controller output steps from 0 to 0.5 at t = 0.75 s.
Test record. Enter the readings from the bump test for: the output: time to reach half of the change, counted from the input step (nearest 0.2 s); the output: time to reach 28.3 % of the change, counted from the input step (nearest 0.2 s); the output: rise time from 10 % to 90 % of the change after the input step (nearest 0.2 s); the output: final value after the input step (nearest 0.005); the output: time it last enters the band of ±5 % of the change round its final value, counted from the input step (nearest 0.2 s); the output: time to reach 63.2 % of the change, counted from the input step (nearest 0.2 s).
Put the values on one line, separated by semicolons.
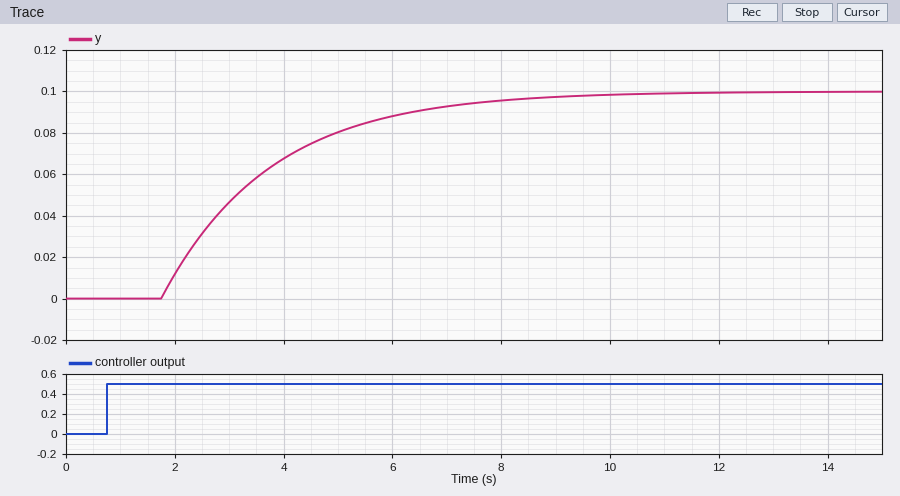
2.4 s; 1.6 s; 4.4 s; 0.100; 7.0 s; 3.0 s
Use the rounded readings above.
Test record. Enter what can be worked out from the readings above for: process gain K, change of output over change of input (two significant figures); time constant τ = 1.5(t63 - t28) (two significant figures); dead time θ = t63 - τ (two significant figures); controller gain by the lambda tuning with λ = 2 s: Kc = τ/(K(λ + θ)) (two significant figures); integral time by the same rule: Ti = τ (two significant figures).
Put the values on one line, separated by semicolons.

0.20; 2.1 s; 0.90 s; 3.6; 2.1 s
